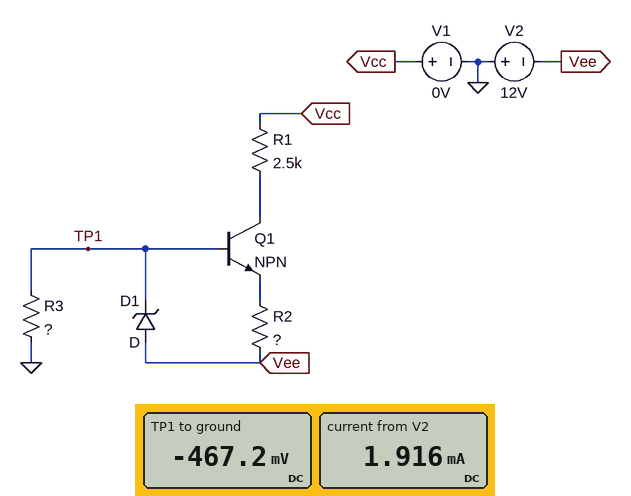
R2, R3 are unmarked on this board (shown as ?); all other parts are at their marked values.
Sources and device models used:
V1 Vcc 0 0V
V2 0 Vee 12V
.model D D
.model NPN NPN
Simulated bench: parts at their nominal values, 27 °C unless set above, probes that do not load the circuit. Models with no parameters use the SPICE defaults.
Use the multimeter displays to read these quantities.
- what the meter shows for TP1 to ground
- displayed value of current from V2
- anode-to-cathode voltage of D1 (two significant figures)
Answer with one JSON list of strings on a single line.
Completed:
["-467.2 mV", "1.916 mA", "-12 V"]
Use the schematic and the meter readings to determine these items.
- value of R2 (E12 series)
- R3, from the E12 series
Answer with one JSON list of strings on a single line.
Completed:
["5.6 kΩ", "330 Ω"]
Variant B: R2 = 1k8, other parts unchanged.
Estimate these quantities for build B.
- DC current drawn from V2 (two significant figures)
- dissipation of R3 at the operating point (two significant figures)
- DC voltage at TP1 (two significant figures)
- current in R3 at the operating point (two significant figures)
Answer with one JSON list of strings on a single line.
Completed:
["5.4 mA", "6.6 mW", "-1.5 V", "4.5 mA"]
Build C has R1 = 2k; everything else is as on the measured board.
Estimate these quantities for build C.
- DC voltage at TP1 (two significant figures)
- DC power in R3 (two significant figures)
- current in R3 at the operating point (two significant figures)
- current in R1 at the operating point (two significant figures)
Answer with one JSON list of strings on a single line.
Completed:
["-430 mV", "570 µW", "1.3 mA", "610 µA"]
